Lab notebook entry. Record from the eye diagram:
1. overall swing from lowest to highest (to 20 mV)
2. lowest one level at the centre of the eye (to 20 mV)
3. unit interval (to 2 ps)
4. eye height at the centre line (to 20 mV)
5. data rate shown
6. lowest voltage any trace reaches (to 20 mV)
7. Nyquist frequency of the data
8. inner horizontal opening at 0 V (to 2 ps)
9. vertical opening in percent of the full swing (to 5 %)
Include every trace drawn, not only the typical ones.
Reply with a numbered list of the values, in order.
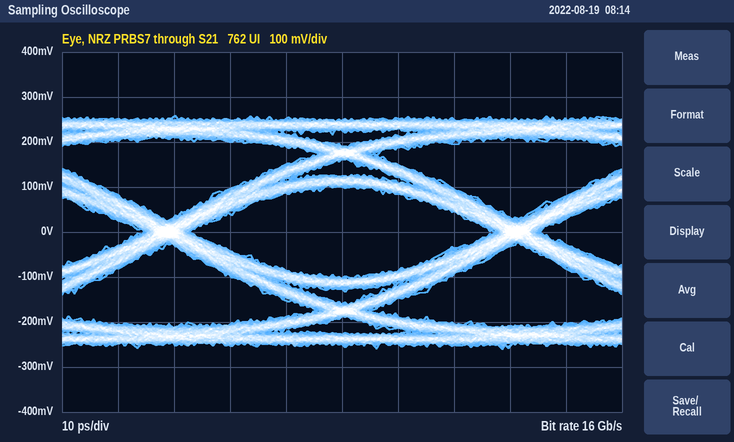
1. 520 mV
2. 100 mV
3. 62 ps
4. 200 mV
5. 16 Gb/s
6. -260 mV
7. 8 GHz
8. 54 ps
9. 40 %
